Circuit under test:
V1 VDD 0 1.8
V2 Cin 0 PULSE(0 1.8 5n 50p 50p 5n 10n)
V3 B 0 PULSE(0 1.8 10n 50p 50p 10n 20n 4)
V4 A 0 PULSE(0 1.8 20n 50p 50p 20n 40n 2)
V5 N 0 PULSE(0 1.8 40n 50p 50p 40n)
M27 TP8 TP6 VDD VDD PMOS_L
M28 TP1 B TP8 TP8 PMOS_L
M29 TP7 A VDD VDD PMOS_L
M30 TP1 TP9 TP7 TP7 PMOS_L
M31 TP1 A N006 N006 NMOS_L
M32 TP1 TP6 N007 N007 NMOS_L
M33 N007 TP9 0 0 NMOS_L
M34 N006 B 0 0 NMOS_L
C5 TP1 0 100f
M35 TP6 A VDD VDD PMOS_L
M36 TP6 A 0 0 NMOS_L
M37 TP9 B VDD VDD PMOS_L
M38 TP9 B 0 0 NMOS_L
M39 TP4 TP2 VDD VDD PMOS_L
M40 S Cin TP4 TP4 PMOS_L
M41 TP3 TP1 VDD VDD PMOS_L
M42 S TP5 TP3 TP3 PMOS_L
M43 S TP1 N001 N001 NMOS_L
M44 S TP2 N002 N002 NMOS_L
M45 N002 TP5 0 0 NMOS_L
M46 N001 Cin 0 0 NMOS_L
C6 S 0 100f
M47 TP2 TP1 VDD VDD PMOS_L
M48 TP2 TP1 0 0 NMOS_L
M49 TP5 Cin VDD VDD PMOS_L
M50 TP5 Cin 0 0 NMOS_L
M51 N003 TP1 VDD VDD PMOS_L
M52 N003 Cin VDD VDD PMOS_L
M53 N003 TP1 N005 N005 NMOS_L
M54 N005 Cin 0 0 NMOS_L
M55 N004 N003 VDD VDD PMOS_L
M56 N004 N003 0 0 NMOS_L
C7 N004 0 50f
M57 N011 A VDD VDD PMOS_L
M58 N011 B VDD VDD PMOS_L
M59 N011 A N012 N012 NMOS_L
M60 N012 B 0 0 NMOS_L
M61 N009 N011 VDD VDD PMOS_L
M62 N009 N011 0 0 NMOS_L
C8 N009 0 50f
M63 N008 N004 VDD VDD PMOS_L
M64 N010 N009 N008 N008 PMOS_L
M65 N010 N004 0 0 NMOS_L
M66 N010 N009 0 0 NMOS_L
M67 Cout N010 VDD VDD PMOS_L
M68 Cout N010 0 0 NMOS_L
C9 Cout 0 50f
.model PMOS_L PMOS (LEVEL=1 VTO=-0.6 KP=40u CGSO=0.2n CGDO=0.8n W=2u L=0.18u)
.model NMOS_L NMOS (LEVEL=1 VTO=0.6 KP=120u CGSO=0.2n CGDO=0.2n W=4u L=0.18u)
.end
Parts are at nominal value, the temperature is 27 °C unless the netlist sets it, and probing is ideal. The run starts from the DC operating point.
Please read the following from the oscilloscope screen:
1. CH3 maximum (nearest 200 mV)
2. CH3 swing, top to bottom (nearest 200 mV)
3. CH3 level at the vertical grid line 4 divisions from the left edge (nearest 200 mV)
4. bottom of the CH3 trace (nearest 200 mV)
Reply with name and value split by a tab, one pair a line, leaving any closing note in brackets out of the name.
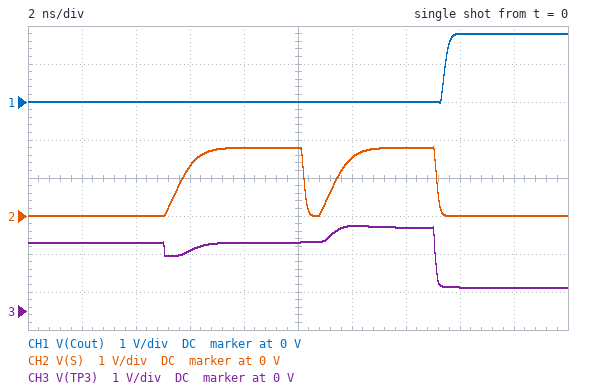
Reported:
CH3 maximum	2.2 V
CH3 swing, top to bottom	1.6 V
CH3 level at the vertical grid line 4 divisions from the left edge	1.8 V
bottom of the CH3 trace	600 mV
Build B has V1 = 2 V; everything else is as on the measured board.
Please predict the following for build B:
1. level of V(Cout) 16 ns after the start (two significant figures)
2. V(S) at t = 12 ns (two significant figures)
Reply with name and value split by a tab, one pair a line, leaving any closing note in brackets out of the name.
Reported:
level of V(Cout) 16 ns after the start	2.0 V
V(S) at t = 12 ns	1.9 V
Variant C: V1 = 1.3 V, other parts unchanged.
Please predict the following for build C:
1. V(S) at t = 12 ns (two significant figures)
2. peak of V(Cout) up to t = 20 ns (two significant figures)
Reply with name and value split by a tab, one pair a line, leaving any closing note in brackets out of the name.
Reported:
V(S) at t = 12 ns	83 mV
peak of V(Cout) up to t = 20 ns	1.3 V
